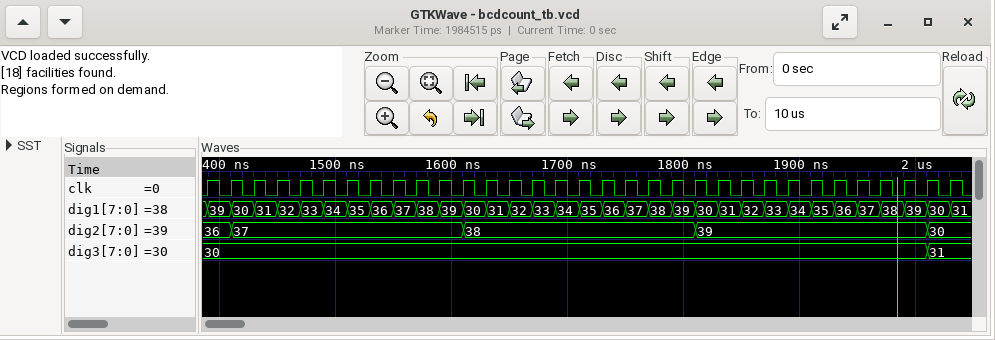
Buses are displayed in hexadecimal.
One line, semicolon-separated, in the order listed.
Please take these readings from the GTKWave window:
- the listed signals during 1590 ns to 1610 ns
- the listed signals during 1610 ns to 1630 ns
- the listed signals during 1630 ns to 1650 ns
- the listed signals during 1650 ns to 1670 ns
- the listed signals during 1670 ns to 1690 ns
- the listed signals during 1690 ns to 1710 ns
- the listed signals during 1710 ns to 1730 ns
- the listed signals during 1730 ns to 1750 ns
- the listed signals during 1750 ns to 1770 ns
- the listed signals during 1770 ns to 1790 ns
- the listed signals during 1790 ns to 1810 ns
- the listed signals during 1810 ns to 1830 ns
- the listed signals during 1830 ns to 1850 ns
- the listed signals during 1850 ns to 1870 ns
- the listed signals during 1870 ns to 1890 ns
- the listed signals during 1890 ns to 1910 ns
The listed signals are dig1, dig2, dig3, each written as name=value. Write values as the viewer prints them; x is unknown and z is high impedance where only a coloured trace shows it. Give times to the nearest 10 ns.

dig1=39, dig2=37, dig3=30; dig1=30, dig2=38, dig3=30; dig1=31, dig2=38, dig3=30; dig1=32, dig2=38, dig3=30; dig1=33, dig2=38, dig3=30; dig1=34, dig2=38, dig3=30; dig1=35, dig2=38, dig3=30; dig1=36, dig2=38, dig3=30; dig1=37, dig2=38, dig3=30; dig1=38, dig2=38, dig3=30; dig1=39, dig2=38, dig3=30; dig1=30, dig2=39, dig3=30; dig1=31, dig2=39, dig3=30; dig1=32, dig2=39, dig3=30; dig1=33, dig2=39, dig3=30; dig1=34, dig2=39, dig3=30
